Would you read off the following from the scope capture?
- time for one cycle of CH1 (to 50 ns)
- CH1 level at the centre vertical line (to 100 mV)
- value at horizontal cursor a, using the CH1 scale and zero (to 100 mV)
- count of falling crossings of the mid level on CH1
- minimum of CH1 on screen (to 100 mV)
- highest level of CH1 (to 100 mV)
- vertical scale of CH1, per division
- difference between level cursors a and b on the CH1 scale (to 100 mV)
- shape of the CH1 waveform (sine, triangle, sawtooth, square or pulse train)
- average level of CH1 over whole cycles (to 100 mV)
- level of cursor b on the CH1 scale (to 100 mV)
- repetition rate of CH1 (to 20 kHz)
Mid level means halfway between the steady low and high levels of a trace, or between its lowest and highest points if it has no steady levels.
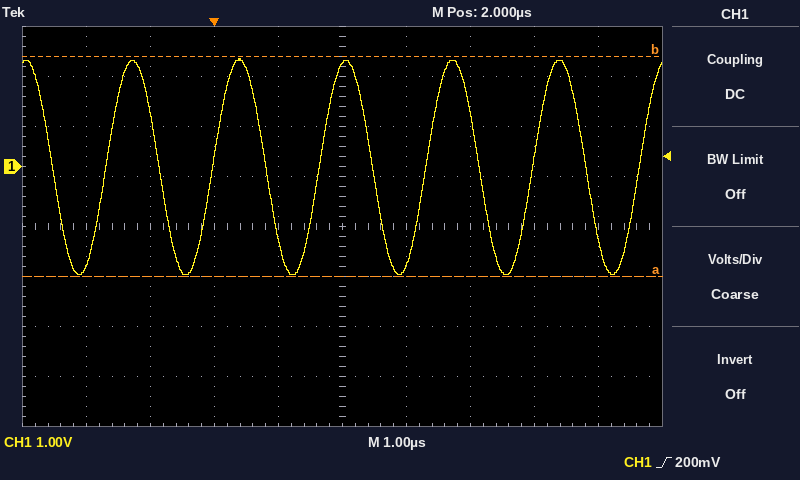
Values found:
1.65 µs
2.0 V
-2.2 V
6
-2.2 V
2.2 V
1 V
4.4 V
sine
0.0 V
2.2 V
600 kHz
